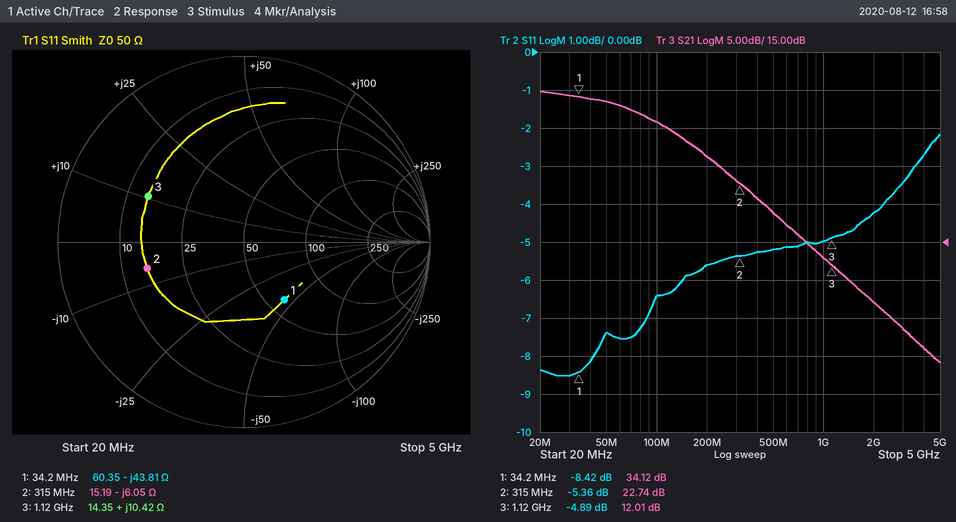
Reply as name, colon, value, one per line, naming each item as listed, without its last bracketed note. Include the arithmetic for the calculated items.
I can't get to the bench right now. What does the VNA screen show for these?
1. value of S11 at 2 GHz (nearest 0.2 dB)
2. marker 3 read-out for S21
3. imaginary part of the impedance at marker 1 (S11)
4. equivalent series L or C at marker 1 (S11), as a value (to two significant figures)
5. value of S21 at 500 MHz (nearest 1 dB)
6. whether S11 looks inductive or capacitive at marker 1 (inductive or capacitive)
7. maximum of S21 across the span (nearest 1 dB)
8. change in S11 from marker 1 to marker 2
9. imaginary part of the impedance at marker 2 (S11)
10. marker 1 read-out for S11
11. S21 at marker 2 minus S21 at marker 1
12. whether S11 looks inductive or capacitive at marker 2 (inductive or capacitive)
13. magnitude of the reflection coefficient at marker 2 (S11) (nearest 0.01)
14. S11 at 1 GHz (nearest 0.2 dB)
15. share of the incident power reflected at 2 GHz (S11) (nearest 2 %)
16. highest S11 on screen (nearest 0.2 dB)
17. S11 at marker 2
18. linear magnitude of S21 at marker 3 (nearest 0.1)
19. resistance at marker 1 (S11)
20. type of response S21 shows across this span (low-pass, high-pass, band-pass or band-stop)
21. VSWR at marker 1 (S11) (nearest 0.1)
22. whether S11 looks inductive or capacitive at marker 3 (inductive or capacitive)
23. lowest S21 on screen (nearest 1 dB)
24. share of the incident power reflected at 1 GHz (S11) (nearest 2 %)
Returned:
value of S11 at 2 GHz: -4.2 dB
marker 3 read-out for S21: 12.01 dB
imaginary part of the impedance at marker 1: -43.81 Ω
equivalent series L or C at marker 1 (S11), as a value: C = 1/(2π × 34.2 MHz × 43.81 Ω) ≈ 106 pF, so 110 pF to two significant figures
value of S21 at 500 MHz: 19 dB
whether S11 looks inductive or capacitive at marker 1: capacitive
maximum of S21 across the span: 35 dB
change in S11 from marker 1 to marker 2: -5.36 − (-8.42) = 3.06 dB
imaginary part of the impedance at marker 2: -6.05 Ω
marker 1 read-out for S11: -8.42 dB
S21 at marker 2 minus S21 at marker 1: 22.74 − (34.12) = -11.38 dB
whether S11 looks inductive or capacitive at marker 2: capacitive
magnitude of the reflection coefficient at marker 2 (S11): 10^(-5.36/20) ≈ 0.54
S11 at 1 GHz: -5.0 dB
share of the incident power reflected at 2 GHz (S11): 10^(-4.2/10) ≈ 38 %
highest S11 on screen: -2.2 dB
S11 at marker 2: -5.36 dB
linear magnitude of S21 at marker 3: 10^(12.01/20) ≈ 4.0
resistance at marker 1: 60.35 Ω
type of response S21 shows across this span: low-pass
VSWR at marker 1 (S11): 2.2
whether S11 looks inductive or capacitive at marker 3: inductive
lowest S21 on screen: -1 dB
share of the incident power reflected at 1 GHz (S11): 10^(-5/10) ≈ 32 %
